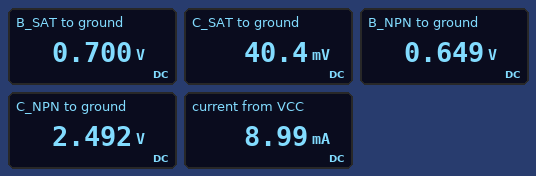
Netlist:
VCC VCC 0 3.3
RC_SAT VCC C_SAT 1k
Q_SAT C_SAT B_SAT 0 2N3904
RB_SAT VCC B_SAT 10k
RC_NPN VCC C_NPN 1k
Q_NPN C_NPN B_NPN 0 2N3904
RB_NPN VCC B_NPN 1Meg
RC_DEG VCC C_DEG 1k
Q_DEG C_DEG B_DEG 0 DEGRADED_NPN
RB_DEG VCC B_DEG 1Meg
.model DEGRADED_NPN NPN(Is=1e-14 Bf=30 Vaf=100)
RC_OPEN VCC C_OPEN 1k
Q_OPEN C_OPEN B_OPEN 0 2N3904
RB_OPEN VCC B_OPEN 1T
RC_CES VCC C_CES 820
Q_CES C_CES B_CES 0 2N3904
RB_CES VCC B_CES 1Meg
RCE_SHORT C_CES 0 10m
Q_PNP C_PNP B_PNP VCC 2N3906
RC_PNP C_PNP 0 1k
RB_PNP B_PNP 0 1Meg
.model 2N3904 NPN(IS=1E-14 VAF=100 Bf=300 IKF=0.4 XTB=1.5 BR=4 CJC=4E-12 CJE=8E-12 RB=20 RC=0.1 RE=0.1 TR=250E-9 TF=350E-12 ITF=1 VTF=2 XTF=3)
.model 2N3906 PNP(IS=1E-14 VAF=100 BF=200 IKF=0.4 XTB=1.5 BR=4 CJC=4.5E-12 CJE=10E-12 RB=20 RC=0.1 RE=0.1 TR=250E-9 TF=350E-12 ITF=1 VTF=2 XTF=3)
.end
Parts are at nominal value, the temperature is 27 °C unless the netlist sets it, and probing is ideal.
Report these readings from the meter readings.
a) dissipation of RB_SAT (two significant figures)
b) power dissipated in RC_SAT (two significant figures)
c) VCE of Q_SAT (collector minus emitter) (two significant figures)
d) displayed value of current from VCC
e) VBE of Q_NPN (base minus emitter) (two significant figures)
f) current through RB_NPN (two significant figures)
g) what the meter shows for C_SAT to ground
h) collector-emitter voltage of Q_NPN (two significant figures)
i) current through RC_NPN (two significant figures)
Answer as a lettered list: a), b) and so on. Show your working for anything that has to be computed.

a) (3.3 V - 700 mV)^2 / 10 kΩ = 680 µW
b) (3.3 V - 40.4 mV)^2 / 1 kΩ = 11 mW
c) 40.4 mV = 40 mV
d) 8.99 mA
e) 649 mV = 650 mV
f) (3.3 V - 649 mV) / 1 MΩ = 2.7 µA
g) 40.4 mV
h) 2.492 V = 2.5 V
i) (3.3 V - 2.492 V) / 1 kΩ = 810 µA
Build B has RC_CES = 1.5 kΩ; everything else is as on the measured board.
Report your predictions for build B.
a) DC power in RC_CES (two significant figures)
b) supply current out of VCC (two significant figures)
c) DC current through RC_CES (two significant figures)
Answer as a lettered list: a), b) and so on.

a) 7.3 mW
b) 7.2 mA
c) 2.2 mA
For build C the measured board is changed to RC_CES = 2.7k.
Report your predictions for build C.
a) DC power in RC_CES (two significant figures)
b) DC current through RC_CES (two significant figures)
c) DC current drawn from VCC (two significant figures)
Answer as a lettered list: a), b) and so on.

a) 4.0 mW
b) 1.2 mA
c) 6.2 mA
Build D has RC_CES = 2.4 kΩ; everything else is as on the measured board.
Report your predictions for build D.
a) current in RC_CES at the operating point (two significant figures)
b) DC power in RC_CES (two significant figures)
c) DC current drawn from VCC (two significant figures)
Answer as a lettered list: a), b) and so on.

a) 1.4 mA
b) 4.5 mW
c) 6.3 mA
